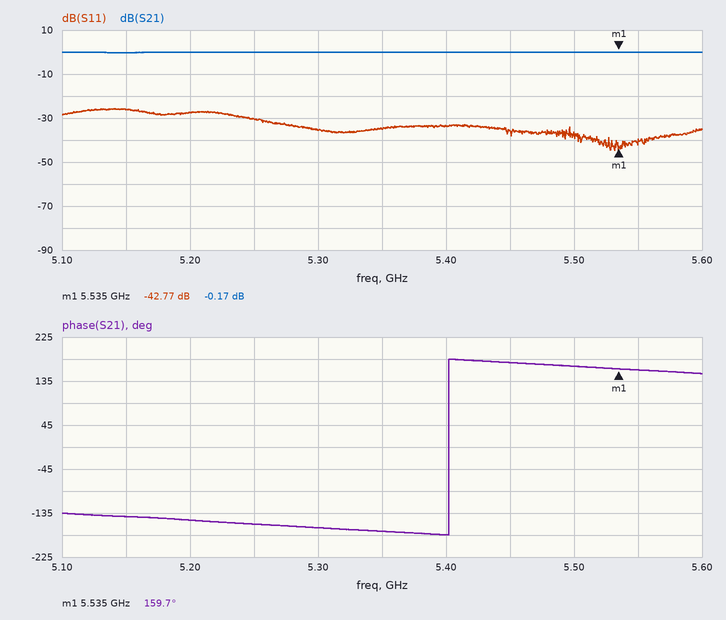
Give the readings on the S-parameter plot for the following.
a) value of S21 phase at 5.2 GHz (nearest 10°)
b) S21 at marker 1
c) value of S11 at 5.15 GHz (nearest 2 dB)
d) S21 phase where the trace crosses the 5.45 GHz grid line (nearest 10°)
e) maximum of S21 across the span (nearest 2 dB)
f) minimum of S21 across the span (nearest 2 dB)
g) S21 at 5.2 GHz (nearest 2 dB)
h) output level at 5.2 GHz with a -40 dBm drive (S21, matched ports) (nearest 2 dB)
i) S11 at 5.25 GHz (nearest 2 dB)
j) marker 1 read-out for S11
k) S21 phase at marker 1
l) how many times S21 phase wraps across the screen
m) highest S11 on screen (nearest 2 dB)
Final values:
-150°
-0.17 dB
-26 dB
170°
0 dB
0 dB
0 dB
-40 dBm
-30 dB
-42.77 dB
159.7°
1
-26 dB
